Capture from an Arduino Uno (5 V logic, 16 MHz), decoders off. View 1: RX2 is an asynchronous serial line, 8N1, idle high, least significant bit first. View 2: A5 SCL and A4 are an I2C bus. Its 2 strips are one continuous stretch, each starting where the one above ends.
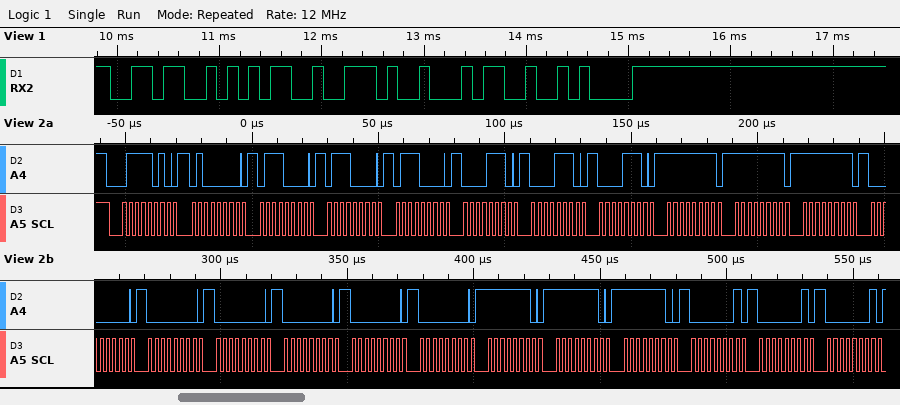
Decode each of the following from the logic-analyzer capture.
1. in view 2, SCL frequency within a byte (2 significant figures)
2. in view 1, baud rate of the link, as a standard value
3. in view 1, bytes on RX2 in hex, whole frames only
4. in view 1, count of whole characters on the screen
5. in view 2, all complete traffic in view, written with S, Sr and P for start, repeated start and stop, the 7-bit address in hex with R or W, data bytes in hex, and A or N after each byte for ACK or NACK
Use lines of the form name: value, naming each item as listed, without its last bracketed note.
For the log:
in view 2, SCL frequency within a byte: 400 kHz
in view 1, baud rate of the link, as a standard value: 9600 baud
in view 1, bytes on RX2 in hex, whole frames only: 36 35 2E 34 0A
in view 1, count of whole characters on the screen: 5
in view 2, all complete traffic in view, written with S, Sr and P for start, repeated start and stop, the 7-bit address in hex with R or W, data bytes in hex, and A or N after each byte for ACK or NACK: S 3DW A 40 A 70 A 70 A 70 A 0E A 0E A 0E A FF A FF A FF A 00 A 00 A 00 A 00 A 00 A 00 A FE A FE A FE A 01 A 01 A 01 A
